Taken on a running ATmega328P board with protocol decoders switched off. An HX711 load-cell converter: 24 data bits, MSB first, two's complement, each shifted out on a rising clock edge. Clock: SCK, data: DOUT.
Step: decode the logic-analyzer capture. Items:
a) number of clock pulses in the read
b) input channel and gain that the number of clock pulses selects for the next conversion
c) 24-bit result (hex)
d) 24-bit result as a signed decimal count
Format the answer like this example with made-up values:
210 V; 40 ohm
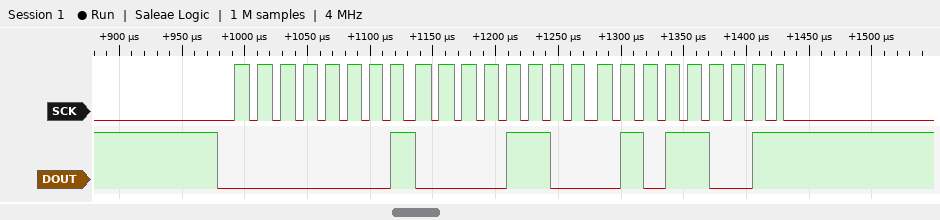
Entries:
25; channel A, gain 128; 0x010C59; 68697
